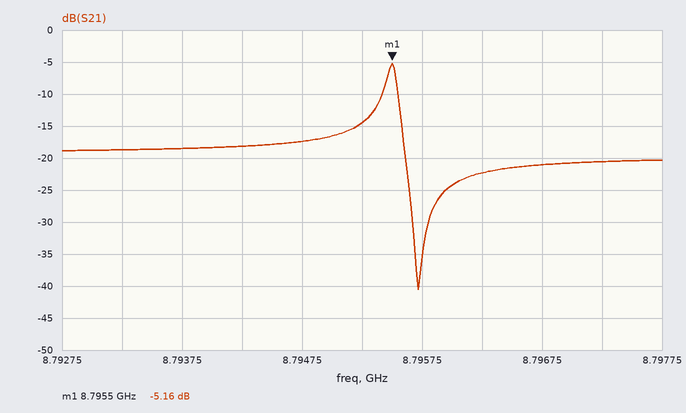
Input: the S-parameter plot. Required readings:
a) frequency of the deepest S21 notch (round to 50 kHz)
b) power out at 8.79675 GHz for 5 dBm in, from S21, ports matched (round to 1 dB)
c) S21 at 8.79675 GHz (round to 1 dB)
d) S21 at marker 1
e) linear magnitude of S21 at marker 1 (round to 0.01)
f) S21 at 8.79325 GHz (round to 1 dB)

8.79570 GHz
-16 dBm
-21 dB
-5.16 dB
0.55
-19 dB
